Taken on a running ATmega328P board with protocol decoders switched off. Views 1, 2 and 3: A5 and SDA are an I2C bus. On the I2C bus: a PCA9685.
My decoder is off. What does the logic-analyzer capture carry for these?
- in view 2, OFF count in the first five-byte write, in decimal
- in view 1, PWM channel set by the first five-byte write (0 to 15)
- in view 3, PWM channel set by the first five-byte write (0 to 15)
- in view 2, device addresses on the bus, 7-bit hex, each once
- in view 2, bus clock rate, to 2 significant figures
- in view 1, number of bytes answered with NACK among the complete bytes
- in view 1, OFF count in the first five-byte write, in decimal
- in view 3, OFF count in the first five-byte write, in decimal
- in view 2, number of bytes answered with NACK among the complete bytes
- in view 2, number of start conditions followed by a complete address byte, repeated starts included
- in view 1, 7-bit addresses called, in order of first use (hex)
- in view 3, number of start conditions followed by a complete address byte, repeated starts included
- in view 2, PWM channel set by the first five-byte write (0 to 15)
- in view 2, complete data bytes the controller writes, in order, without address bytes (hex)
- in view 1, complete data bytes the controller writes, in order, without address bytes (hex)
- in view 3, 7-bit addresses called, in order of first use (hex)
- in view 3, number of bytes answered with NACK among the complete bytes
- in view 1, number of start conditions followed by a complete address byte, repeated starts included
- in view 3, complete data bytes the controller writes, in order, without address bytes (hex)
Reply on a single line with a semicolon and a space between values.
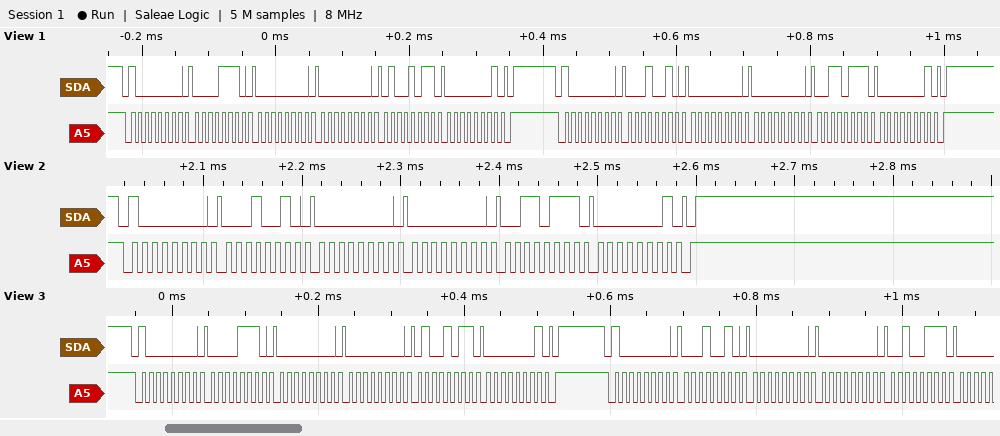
311; 2; 2; 0x40; 100 kHz; 0; 331; 331; 0; 1; 0x40; 2; 3; 12 00 00 37 01; 0E 00 00 4B 01 12 00 00 37 01; 0x40; 0; 2; 0E 00 00 4B 01 12 00 00 27
